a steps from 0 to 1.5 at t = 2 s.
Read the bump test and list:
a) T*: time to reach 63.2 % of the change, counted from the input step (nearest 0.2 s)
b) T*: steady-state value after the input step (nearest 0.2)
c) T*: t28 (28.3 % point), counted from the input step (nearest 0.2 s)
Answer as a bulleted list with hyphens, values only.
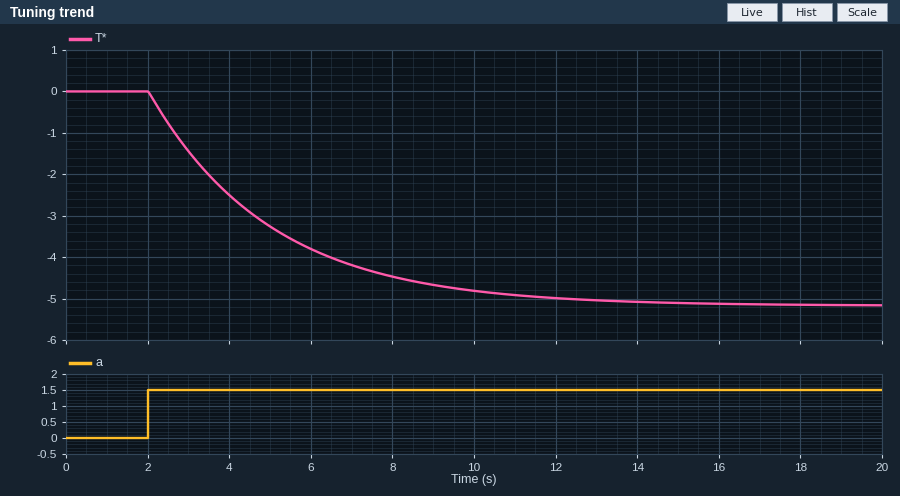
- 3.0 s
- -5.2
- 1.0 s
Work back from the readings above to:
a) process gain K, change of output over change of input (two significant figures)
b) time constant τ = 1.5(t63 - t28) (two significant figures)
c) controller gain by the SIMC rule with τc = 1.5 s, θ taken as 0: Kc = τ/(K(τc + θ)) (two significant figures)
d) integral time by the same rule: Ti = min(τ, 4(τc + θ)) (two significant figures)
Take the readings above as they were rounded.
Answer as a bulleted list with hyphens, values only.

- -3.5
- 3.0 s
- -0.57
- 3.0 s
